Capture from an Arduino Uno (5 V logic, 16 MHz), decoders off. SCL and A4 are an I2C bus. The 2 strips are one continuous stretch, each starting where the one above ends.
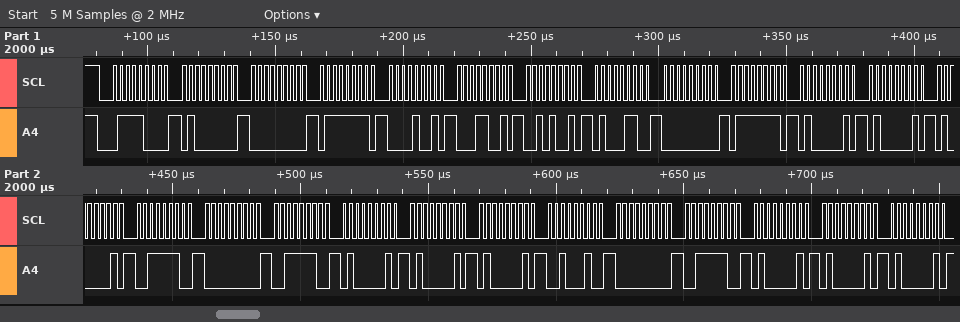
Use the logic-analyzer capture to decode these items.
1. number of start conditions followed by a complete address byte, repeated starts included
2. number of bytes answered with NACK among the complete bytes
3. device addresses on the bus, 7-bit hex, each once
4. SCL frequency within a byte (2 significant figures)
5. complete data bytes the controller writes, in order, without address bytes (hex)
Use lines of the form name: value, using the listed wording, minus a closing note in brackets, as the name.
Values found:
number of start conditions followed by a complete address byte, repeated starts included: 1
number of bytes answered with NACK among the complete bytes: 0
device addresses on the bus, 7-bit hex, each once: 0x3C
SCL frequency within a byte: 400 kHz
complete data bytes the controller writes, in order, without address bytes: 40 00 7F 09 19 29 46 00 7F 41 41 41 3E 00 3E 41 41 41 22 00 3E 41 41 41
